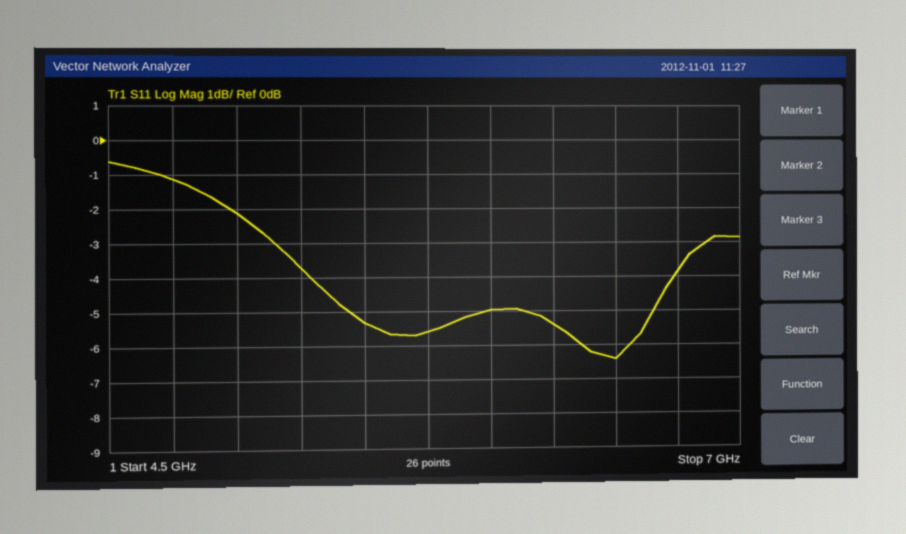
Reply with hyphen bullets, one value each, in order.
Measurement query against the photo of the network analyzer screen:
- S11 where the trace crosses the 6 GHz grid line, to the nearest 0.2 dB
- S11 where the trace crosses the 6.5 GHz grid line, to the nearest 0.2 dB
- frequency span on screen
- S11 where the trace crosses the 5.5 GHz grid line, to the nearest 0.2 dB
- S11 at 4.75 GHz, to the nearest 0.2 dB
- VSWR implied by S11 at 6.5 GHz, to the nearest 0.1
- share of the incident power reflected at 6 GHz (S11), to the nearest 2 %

- -5.0 dB
- -6.4 dB
- 2.5 GHz
- -5.4 dB
- -1.2 dB
- 2.8
- 32 %
